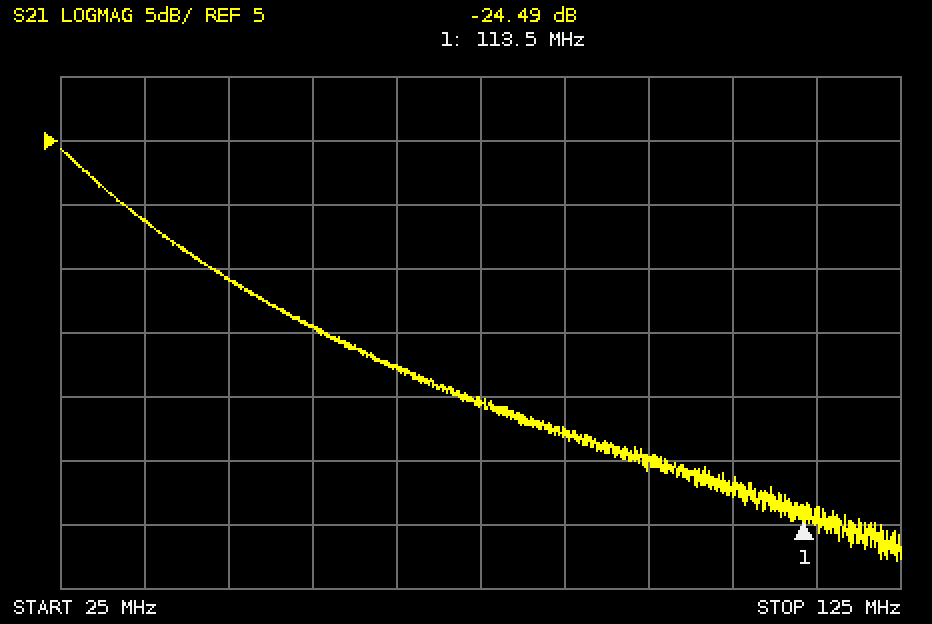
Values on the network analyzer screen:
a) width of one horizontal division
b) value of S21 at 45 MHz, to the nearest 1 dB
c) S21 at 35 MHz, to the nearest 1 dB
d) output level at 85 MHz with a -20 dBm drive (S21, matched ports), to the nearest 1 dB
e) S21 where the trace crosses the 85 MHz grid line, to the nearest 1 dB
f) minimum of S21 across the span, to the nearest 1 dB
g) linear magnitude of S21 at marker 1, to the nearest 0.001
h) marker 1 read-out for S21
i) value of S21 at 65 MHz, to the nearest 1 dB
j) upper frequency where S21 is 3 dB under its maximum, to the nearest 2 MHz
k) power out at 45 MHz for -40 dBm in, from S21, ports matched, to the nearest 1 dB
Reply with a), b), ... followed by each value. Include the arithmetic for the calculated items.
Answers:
a) 10 MHz
b) -6 dB
c) -1 dB
d) -20 dBm + (-18 dB) = -38 dBm
e) -18 dB
f) -28 dB
g) 10^(-24.49/20) ≈ 0.060
h) -24.49 dB
i) -13 dB
j) 30 MHz
k) -40 dBm + (-6 dB) = -46 dBm
